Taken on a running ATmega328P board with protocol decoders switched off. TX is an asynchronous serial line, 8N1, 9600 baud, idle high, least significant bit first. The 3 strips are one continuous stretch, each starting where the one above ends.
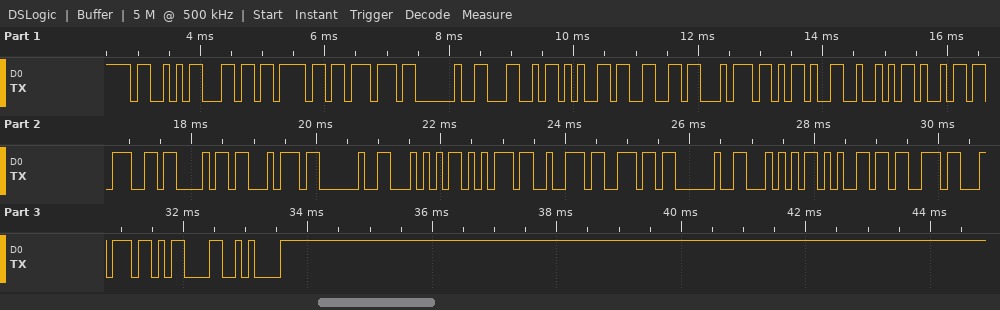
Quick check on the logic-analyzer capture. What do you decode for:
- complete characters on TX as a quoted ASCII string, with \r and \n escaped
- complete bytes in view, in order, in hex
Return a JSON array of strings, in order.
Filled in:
["\"Slow Left-Right Turn Test\\r\\n\"", "53 6C 6F 77 20 4C 65 66 74 2D 52 69 67 68 74 20 54 75 72 6E 20 54 65 73 74 0D 0A"]
